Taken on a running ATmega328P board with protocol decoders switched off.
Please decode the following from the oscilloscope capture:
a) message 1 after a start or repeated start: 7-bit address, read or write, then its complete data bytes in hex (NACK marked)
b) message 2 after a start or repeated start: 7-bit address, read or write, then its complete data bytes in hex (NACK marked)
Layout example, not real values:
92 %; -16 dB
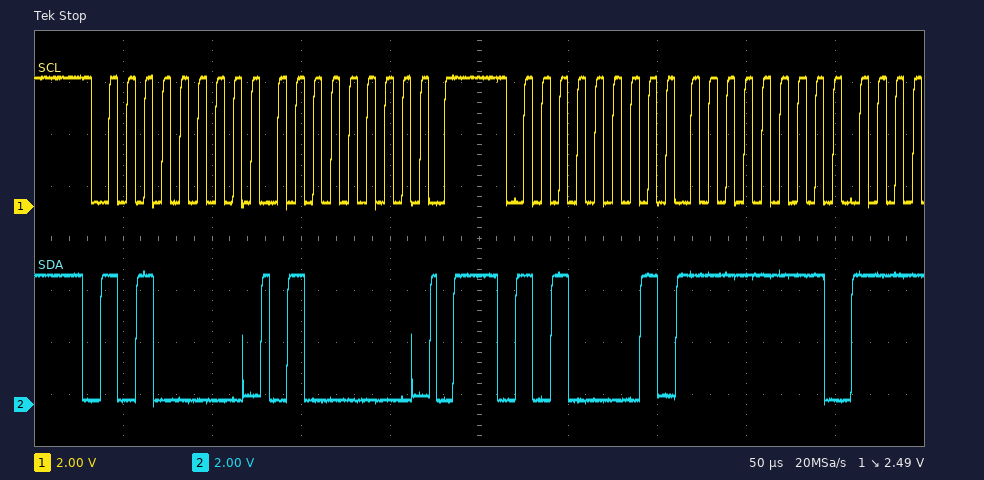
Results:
0x50 write: 40; 0x50 read: FF
